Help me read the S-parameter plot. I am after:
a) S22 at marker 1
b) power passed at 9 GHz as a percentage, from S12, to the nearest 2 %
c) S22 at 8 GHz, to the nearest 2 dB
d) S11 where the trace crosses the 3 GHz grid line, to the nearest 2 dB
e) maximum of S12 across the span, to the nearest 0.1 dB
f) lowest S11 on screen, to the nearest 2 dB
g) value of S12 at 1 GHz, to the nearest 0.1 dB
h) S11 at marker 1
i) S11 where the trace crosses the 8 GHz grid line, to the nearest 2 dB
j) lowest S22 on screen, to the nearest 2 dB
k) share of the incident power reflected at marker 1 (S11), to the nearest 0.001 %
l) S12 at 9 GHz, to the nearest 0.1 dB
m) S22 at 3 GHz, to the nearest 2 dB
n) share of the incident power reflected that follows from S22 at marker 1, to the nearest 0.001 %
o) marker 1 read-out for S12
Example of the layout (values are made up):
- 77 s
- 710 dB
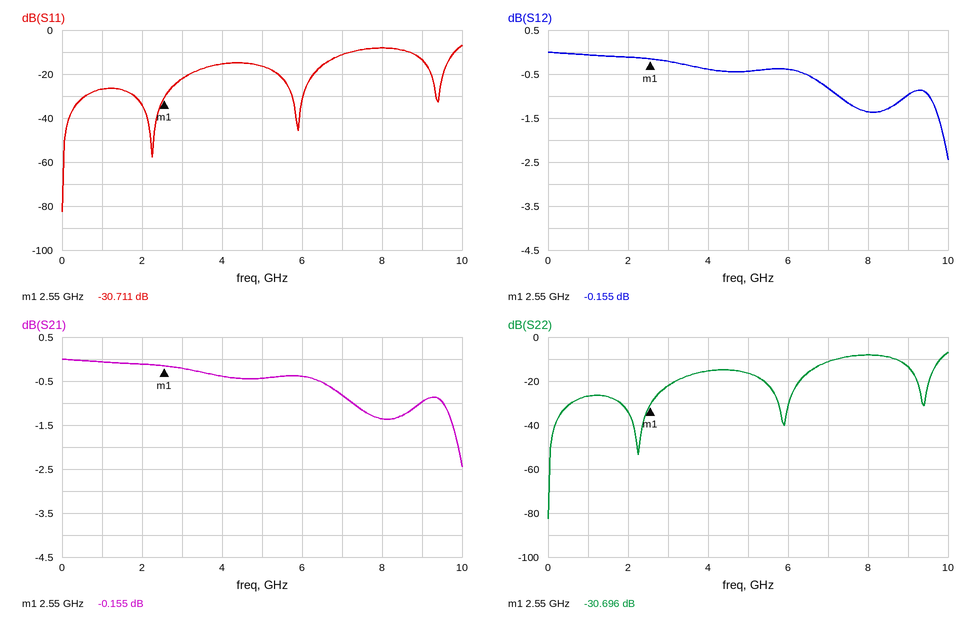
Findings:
- -30.696 dB
- 80 %
- -8 dB
- -22 dB
- 0.0 dB
- -82 dB
- -0.1 dB
- -30.711 dB
- -8 dB
- -82 dB
- 0.085 %
- -1.0 dB
- -22 dB
- 0.085 %
- -0.155 dB
